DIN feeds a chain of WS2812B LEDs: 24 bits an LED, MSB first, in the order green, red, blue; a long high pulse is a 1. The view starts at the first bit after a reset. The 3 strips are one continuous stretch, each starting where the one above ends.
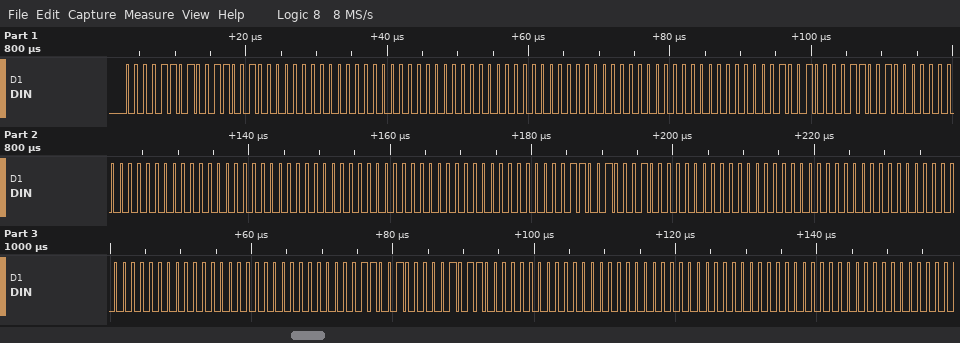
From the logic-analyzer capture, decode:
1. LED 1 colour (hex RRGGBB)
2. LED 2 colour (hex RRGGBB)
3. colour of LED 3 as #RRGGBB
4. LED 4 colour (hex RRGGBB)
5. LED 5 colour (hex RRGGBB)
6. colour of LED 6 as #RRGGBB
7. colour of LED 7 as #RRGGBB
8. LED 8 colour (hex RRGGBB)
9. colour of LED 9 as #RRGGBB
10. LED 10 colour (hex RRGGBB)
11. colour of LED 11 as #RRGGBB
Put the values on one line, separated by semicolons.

#320D00; #000000; #000000; #322400; #000000; #000000; #203200; #000000; #000000; #0B3200; #000000
